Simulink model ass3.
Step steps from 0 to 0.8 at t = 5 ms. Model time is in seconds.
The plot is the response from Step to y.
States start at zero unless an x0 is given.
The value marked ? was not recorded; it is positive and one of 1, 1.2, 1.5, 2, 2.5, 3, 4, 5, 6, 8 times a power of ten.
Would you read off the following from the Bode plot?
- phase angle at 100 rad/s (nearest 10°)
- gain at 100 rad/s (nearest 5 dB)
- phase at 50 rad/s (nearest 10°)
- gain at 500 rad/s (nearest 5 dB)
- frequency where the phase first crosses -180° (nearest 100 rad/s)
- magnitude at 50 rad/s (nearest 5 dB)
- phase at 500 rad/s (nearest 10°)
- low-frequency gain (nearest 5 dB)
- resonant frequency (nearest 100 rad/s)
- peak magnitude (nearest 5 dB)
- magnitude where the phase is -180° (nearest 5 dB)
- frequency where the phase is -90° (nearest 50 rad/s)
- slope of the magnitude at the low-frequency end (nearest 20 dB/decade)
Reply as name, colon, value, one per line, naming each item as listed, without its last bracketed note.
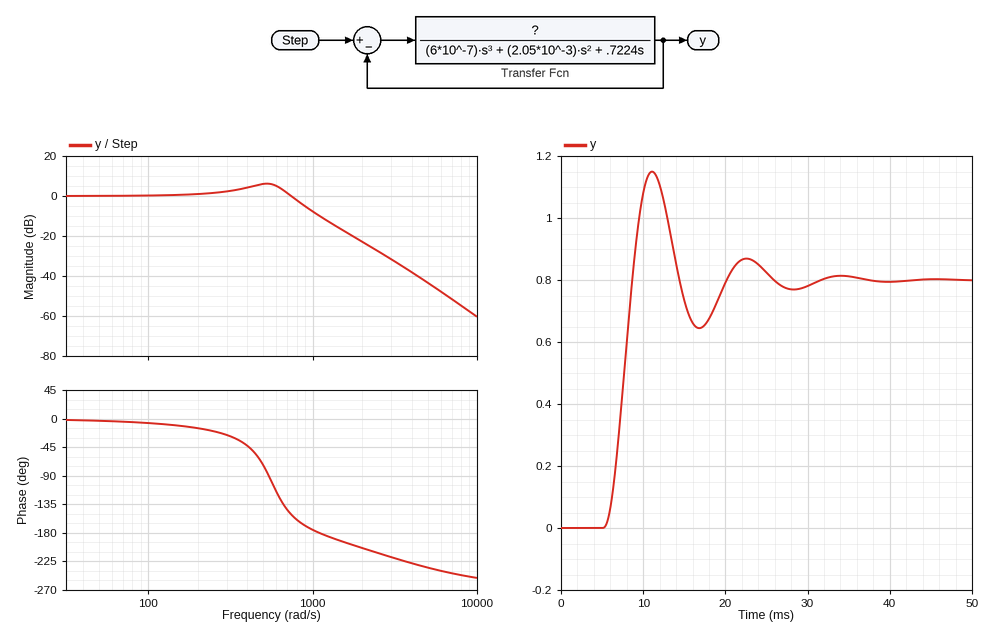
phase angle at 100 rad/s: -10°
gain at 100 rad/s: 0 dB
phase at 50 rad/s: 0°
gain at 500 rad/s: 5 dB
frequency where the phase first crosses -180°: 1100 rad/s
magnitude at 50 rad/s: 0 dB
phase at 500 rad/s: -70°
low-frequency gain: 0 dB
resonant frequency: 500 rad/s
peak magnitude: 5 dB
magnitude where the phase is -180°: -10 dB
frequency where the phase is -90°: 550 rad/s
slope of the magnitude at the low-frequency end: 0 dB/decade
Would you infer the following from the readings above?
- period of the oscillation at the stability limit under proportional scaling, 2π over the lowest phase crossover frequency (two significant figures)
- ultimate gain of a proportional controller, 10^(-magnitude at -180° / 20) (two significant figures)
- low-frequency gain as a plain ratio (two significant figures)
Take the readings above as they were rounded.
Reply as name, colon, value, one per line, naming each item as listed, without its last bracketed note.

period of the oscillation at the stability limit under proportional scaling, 2π over the lowest phase crossover frequency: 0.0057 s
ultimate gain of a proportional controller, 10^(-magnitude at -180° / 20): 3.2
low-frequency gain as a plain ratio: 1.0
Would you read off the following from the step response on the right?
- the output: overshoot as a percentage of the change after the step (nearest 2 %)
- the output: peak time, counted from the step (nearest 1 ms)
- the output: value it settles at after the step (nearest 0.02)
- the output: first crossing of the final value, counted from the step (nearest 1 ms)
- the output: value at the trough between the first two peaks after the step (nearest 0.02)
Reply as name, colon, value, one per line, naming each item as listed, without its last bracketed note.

the output: overshoot as a percentage of the change after the step: 44 %
the output: peak time, counted from the step: 6 ms
the output: value it settles at after the step: 0.80
the output: first crossing of the final value, counted from the step: 4 ms
the output: value at the trough between the first two peaks after the step: 0.64
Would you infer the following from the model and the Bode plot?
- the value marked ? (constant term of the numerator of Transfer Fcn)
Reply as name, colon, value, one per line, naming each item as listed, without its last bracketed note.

the value marked ?: 600
